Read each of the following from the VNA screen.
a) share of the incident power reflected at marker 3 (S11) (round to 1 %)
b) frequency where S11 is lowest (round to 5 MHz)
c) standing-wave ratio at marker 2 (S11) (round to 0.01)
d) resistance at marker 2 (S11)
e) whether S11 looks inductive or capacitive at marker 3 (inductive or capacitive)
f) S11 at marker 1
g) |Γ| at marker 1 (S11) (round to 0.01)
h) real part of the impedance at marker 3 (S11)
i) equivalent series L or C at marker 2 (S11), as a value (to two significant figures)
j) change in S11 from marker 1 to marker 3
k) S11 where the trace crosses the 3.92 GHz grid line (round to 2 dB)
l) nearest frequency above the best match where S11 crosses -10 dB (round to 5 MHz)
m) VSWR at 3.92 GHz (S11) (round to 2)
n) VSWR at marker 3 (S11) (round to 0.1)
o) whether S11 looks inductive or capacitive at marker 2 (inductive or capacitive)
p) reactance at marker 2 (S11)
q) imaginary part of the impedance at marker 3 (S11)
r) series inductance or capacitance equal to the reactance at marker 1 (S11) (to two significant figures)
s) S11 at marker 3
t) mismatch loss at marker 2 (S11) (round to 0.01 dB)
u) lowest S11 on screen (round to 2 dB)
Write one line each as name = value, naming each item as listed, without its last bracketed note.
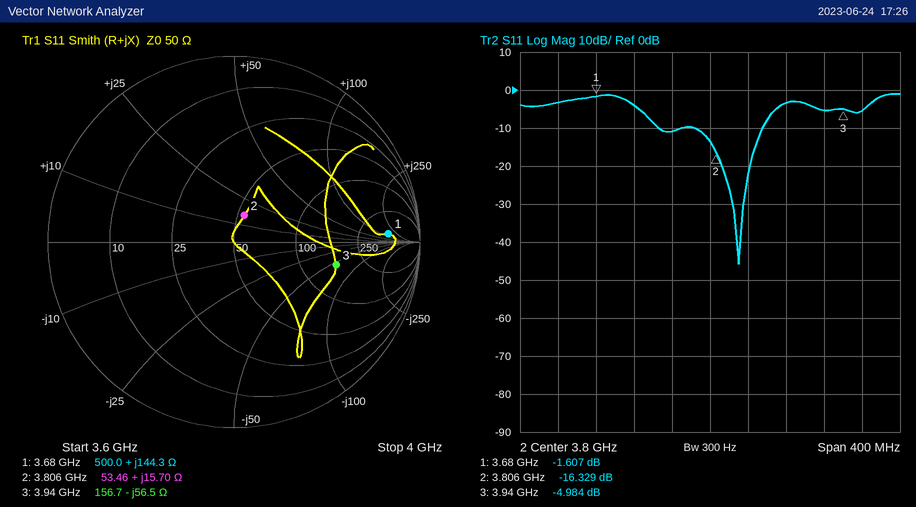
share of the incident power reflected at marker 3 (S11) = 32 %
frequency where S11 is lowest = 3.830 GHz
standing-wave ratio at marker 2 (S11) = 1.36
resistance at marker 2 = 53.46 Ω
whether S11 looks inductive or capacitive at marker 3 = capacitive
S11 at marker 1 = -1.607 dB
|Γ| at marker 1 (S11) = 0.83
real part of the impedance at marker 3 = 156.7 Ω
equivalent series L or C at marker 2 (S11), as a value = 660 pH
change in S11 from marker 1 to marker 3 = -3.377 dB
S11 where the trace crosses the 3.92 GHz grid line = -6 dB
nearest frequency above the best match where S11 crosses -10 dB = 3.855 GHz
VSWR at 3.92 GHz (S11) = 4
VSWR at marker 3 (S11) = 3.6
whether S11 looks inductive or capacitive at marker 2 = inductive
reactance at marker 2 = +15.70 Ω
imaginary part of the impedance at marker 3 = -56.5 Ω
series inductance or capacitance equal to the reactance at marker 1 (S11) = 6.2 nH
S11 at marker 3 = -4.984 dB
mismatch loss at marker 2 (S11) = 0.10 dB
lowest S11 on screen = -46 dB
